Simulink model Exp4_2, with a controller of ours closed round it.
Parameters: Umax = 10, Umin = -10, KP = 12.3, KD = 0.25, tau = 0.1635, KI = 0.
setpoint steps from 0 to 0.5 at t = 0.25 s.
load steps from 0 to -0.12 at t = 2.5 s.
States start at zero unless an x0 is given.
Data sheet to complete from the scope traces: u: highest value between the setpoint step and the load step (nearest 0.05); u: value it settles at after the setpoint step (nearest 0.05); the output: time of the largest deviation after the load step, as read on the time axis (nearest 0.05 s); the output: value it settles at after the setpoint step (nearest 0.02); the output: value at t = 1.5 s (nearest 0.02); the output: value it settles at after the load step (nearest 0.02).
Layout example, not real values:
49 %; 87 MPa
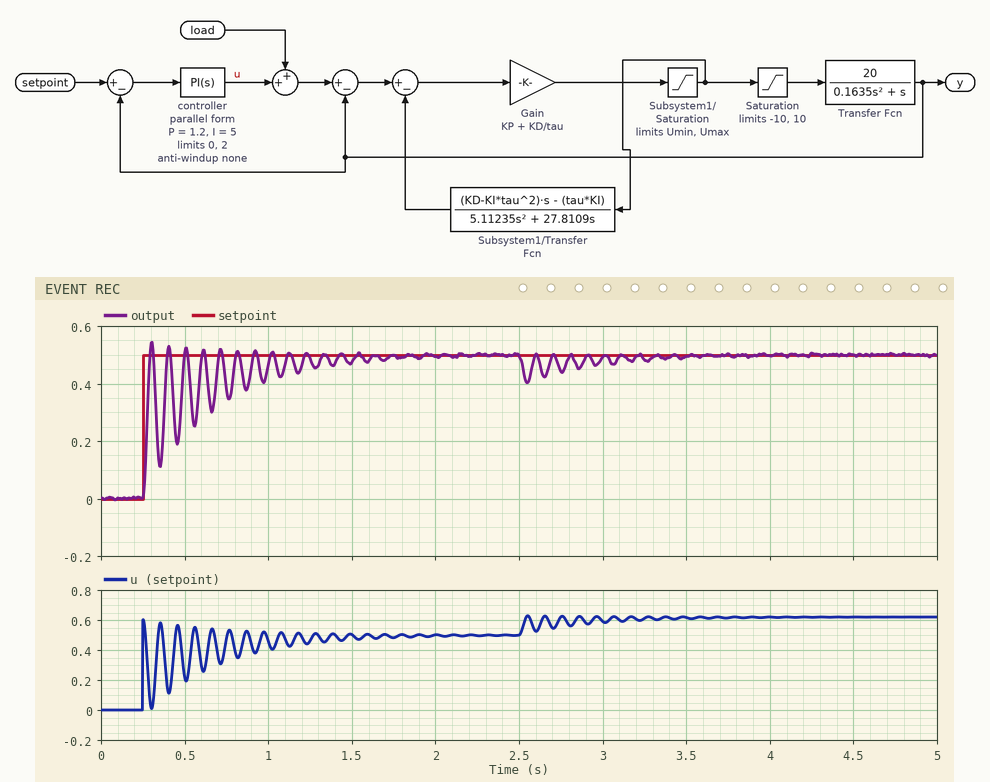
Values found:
0.60; 0.50; 2.55 s; 0.50; 0.48; 0.50
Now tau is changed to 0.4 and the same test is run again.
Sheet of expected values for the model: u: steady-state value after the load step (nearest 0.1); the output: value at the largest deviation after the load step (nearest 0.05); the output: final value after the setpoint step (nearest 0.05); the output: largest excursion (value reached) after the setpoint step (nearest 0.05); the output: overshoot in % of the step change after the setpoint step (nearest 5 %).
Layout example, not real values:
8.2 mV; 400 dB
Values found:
0.6; 0.40; 0.50; 0.55; 10 %
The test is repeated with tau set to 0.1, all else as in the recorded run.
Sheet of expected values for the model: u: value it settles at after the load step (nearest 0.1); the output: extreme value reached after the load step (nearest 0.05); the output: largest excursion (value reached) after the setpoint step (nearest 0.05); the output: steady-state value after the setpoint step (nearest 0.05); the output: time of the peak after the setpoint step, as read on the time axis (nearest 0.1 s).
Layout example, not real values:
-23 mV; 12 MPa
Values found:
0.6; 0.40; 0.55; 0.50; 0.3 s
